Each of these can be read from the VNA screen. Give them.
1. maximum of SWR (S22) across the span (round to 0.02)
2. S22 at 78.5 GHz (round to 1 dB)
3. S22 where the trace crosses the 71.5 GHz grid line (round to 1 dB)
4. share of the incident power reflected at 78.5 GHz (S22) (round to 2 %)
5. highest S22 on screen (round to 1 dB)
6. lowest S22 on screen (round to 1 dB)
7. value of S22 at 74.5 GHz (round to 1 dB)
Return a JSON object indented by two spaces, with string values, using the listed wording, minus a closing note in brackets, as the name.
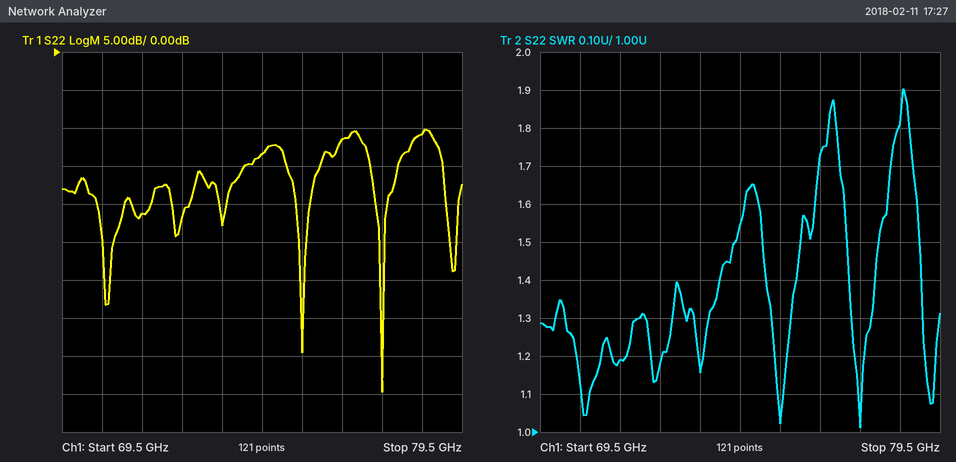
{
  "maximum of SWR (S22) across the span": "1.90",
  "S22 at 78.5 GHz": "-11 dB",
  "S22 where the trace crosses the 71.5 GHz grid line": "-21 dB",
  "share of the incident power reflected at 78.5 GHz (S22)": "8 %",
  "highest S22 on screen": "-10 dB",
  "lowest S22 on screen": "-45 dB",
  "value of S22 at 74.5 GHz": "-13 dB"
}
